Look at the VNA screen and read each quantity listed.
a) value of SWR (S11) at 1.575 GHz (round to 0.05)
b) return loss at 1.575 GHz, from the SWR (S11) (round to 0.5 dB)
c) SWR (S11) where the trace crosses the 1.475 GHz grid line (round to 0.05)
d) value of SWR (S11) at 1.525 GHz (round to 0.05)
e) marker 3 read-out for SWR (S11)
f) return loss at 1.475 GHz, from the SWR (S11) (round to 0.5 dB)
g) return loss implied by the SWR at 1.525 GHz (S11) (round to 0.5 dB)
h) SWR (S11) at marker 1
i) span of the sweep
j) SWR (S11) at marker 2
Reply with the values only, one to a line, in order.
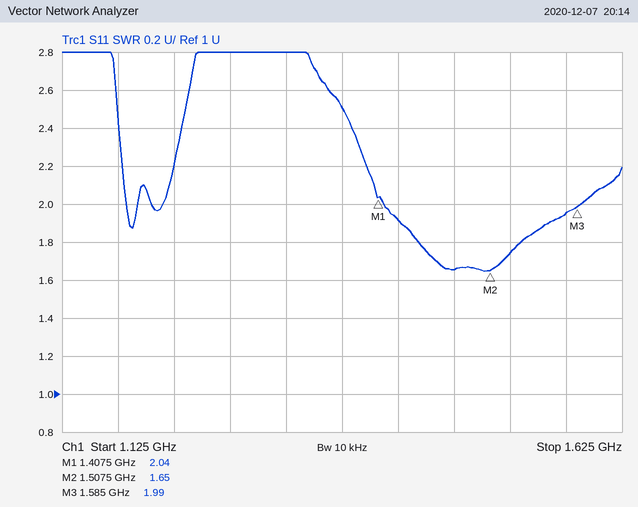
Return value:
1.95
10.0 dB
1.65
1.75
1.99
12.0 dB
11.5 dB
2.04
500 MHz
1.65
